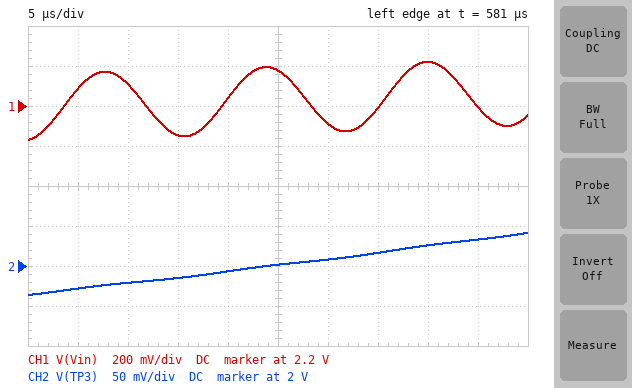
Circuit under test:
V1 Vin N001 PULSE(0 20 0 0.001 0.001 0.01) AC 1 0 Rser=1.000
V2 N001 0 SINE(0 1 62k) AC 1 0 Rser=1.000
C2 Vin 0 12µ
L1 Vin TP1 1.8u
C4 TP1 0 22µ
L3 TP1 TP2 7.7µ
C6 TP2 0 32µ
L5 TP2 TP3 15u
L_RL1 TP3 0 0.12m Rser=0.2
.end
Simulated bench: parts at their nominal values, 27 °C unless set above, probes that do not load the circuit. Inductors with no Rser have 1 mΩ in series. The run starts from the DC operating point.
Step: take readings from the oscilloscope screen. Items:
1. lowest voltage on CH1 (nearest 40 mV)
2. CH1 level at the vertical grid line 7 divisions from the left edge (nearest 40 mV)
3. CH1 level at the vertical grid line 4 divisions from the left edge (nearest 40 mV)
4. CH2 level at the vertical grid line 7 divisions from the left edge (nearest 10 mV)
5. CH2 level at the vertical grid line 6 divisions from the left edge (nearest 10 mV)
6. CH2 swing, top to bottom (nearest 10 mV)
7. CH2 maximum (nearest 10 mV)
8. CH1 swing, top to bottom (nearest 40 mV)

2.04 V
2.20 V
2.24 V
2.02 V
2.01 V
80 mV
2.04 V
400 mV
